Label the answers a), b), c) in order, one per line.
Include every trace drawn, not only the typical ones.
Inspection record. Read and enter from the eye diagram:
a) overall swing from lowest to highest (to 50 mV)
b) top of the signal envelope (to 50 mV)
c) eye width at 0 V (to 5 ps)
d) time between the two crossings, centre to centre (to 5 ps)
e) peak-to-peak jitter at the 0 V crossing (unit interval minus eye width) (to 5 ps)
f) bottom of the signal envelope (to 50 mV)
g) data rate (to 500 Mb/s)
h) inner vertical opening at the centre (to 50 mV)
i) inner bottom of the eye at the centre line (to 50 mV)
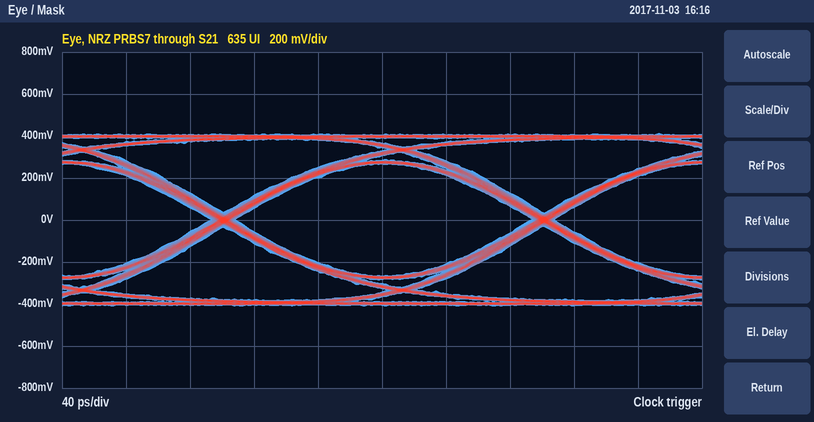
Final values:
a) 800 mV
b) 400 mV
c) 185 ps
d) 200 ps
e) 15 ps
f) -400 mV
g) 5.0 Gb/s
h) 550 mV
i) -250 mV
